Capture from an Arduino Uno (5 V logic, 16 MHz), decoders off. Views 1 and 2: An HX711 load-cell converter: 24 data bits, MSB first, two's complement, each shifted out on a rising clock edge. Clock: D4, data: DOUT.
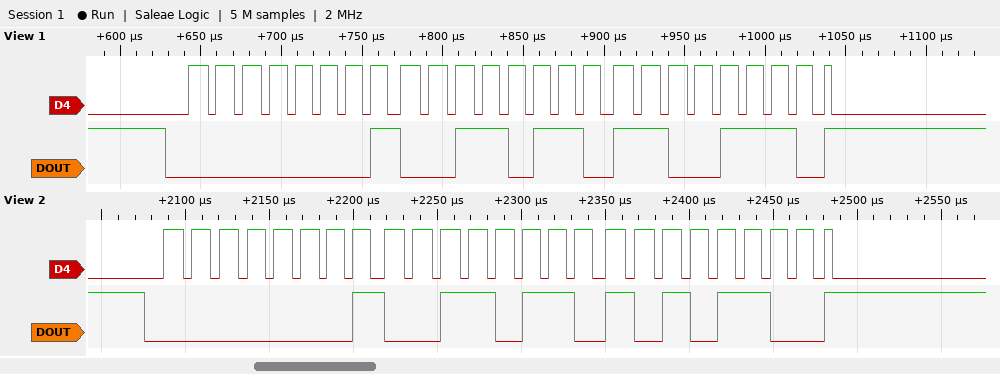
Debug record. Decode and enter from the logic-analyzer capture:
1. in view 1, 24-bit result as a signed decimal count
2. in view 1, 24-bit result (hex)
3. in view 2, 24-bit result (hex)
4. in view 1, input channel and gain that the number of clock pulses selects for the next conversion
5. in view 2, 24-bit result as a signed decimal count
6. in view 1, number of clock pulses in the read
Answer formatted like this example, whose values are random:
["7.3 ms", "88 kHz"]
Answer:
["79566", "0x0136CE", "0x0136AC", "channel A, gain 128", "79532", "25"]
